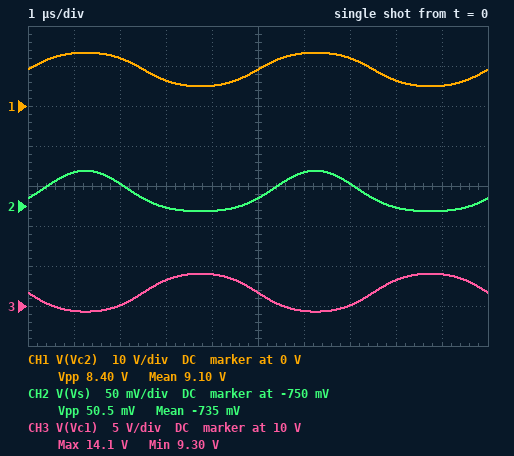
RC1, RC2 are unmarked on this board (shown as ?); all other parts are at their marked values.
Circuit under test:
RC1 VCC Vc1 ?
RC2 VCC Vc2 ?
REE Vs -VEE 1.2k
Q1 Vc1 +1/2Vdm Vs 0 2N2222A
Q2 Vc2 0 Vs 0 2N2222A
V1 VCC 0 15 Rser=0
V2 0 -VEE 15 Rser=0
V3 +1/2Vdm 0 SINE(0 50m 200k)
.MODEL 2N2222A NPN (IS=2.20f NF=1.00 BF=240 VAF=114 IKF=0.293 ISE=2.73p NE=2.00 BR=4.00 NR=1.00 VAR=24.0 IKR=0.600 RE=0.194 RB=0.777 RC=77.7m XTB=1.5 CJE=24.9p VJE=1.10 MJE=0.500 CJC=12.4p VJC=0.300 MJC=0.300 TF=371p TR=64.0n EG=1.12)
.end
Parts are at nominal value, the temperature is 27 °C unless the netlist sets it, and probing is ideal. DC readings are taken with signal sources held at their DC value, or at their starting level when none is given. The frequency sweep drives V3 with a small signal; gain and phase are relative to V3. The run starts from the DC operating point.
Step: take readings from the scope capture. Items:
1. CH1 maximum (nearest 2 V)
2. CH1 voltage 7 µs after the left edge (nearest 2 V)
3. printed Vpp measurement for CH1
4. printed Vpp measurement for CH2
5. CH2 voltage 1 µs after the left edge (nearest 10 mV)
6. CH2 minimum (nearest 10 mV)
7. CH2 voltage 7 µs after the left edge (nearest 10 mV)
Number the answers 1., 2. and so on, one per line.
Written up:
1. 14 V
2. 12 V
3. 8.40 V
4. 50.5 mV
5. -710 mV
6. -760 mV
7. -720 mV
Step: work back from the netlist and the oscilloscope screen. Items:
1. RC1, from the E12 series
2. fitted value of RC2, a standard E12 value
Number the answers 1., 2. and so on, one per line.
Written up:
1. 560 Ω
2. 1 kΩ
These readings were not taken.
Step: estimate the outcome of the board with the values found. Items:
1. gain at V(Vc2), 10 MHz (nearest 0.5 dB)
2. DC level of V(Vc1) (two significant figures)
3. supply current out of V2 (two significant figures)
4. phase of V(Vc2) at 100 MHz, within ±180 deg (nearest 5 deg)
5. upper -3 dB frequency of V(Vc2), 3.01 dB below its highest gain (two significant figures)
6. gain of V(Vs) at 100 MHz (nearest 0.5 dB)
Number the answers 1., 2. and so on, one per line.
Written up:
1. 40.0 dB
2. 12 V
3. 12 mA
4. -75 deg
5. 33 MHz
6. -6.0 dB
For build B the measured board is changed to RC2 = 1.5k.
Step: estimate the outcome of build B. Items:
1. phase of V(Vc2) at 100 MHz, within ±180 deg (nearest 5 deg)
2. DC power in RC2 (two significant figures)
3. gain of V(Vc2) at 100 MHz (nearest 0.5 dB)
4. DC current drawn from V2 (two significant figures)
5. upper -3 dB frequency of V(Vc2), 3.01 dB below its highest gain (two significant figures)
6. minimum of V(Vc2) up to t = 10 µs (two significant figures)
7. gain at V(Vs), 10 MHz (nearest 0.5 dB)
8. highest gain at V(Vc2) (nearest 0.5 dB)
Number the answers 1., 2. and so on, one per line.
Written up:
1. -85 deg
2. 50 mW
3. 29.5 dB
4. 12 mA
5. 20 MHz
6. -20 mV
7. -5.5 dB
8. 43.5 dB
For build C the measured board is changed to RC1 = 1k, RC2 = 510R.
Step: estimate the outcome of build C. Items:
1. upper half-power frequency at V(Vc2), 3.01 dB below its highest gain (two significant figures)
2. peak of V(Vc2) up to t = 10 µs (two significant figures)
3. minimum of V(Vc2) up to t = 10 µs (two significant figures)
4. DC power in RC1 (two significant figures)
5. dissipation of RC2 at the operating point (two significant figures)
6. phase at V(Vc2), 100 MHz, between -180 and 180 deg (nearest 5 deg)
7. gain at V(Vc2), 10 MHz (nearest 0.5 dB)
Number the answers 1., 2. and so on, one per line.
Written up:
1. 65 MHz
2. 14 V
3. 9.8 V
4. 34 mW
5. 18 mW
6. -60 deg
7. 34.5 dB
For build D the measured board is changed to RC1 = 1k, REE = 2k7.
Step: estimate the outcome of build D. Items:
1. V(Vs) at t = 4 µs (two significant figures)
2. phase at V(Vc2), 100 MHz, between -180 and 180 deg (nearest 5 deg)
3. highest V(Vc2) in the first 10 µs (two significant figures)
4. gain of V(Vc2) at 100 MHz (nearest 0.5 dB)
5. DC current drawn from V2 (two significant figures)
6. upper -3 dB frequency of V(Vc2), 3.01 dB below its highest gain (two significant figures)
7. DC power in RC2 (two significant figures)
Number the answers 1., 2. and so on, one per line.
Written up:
1. -730 mV
2. -70 deg
3. 14 V
4. 24.5 dB
5. 5.3 mA
6. 37 MHz
7. 6.9 mW
